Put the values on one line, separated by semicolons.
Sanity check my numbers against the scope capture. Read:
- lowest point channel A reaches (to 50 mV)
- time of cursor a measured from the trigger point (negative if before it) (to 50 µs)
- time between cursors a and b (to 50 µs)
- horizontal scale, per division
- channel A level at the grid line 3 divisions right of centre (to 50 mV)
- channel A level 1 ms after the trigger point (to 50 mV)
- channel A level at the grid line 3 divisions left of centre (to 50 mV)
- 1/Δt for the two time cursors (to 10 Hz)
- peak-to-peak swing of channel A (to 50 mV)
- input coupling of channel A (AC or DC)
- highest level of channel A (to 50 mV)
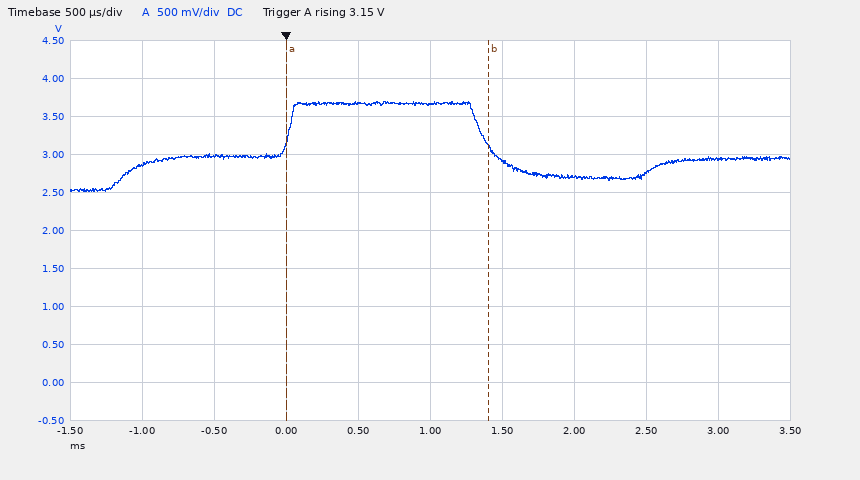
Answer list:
2.50 V; 0 µs; 1.40 ms; 500 µs; 2.75 V; 3.65 V; 3.00 V; 710 Hz; 1.20 V; DC; 3.70 V
